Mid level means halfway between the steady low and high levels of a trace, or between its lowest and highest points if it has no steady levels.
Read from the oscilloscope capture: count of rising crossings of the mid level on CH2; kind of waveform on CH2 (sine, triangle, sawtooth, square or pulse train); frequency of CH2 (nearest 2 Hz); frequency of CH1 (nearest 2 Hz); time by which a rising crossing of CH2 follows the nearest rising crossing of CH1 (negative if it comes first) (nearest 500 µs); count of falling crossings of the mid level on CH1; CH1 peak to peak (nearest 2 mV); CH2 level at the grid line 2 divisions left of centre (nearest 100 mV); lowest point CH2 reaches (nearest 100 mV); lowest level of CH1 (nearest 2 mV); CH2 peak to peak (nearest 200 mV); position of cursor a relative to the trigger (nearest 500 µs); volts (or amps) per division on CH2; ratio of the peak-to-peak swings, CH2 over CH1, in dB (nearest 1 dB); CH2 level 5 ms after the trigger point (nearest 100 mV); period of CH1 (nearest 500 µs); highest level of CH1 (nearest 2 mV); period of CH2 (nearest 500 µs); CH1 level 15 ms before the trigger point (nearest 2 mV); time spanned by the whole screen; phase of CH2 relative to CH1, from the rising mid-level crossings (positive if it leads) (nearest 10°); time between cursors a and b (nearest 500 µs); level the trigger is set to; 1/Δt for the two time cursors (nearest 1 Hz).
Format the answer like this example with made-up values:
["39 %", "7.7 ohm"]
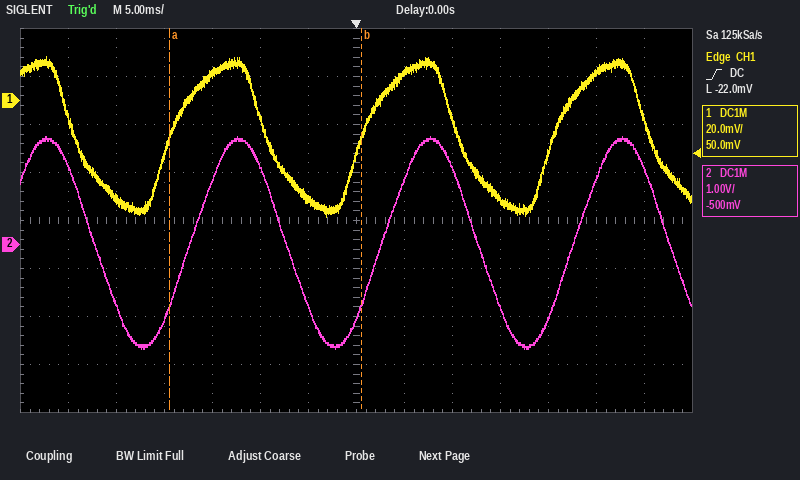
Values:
["3", "sine", "50 Hz", "50 Hz", "+2.0 ms", "4", "66 mV", "1.6 V", "-2.2 V", "-48 mV", "4.4 V", "-19.5 ms", "1 V", "36 dB", "1.3 V", "20.0 ms", "18 mV", "20.0 ms", "12 mV", "70 ms", "-40°", "20.0 ms", "-22.0 mV", "50 Hz"]
